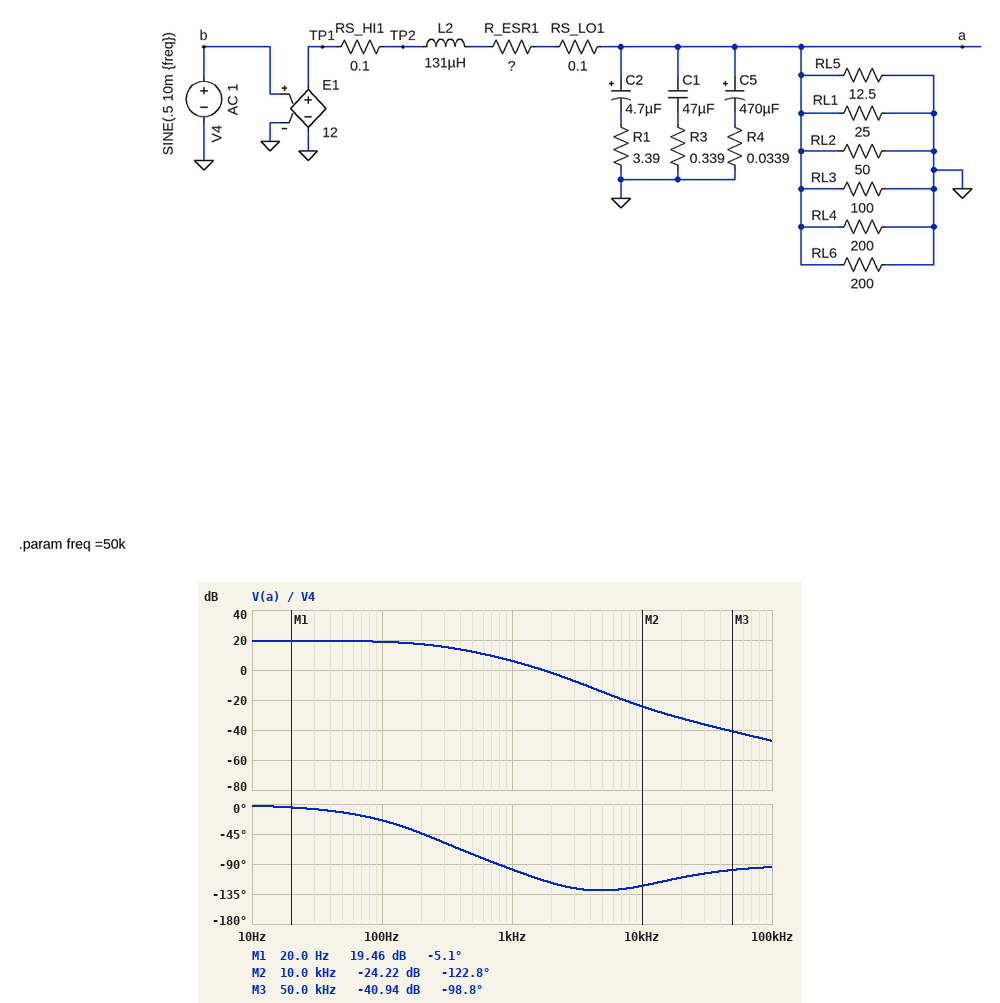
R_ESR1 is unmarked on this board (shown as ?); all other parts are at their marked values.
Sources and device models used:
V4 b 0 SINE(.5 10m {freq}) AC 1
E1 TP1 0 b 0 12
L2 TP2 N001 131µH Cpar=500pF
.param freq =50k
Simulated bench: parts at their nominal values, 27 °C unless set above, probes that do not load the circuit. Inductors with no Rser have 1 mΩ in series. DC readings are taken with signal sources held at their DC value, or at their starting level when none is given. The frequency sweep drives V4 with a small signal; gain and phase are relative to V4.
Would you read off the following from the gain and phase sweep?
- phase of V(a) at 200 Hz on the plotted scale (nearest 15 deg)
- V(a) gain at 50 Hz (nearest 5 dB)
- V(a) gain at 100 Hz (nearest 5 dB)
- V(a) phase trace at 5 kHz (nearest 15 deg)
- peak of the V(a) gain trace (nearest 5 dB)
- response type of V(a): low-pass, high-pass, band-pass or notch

-45 deg
20 dB
20 dB
-135 deg
20 dB
low-pass
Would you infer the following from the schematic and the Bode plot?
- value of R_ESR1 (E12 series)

1.5 Ω
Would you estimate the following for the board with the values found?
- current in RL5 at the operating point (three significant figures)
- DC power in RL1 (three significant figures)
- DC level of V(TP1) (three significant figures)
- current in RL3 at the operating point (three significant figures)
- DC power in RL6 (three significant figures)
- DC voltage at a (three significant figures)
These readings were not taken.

377 mA
890 mW
6.00 V
47.2 mA
111 mW
4.72 V
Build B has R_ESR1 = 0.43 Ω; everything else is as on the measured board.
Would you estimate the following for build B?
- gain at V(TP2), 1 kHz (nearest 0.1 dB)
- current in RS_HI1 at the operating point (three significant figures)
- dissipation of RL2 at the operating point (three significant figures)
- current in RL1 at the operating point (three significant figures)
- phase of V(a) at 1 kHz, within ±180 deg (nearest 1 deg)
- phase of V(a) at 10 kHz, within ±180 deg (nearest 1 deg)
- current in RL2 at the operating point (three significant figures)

20.8 dB
872 mA
594 mW
218 mA
-119 deg
-130 deg
109 mA
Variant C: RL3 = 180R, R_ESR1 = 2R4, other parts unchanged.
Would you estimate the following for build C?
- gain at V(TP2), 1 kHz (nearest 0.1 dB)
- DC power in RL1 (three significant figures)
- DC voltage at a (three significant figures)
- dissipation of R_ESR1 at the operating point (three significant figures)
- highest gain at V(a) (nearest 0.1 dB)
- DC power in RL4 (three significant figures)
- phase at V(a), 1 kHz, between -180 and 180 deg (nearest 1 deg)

21.3 dB
730 mW
4.27 V
1.06 W
18.6 dB
91.2 mW
-93 deg
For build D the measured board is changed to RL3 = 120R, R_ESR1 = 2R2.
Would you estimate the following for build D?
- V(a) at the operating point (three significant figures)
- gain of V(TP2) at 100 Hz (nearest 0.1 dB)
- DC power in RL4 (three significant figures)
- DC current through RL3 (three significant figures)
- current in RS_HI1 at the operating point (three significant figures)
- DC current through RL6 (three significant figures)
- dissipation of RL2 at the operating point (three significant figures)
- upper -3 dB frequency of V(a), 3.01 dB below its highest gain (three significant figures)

4.35 V
21.4 dB
94.5 mW
36.2 mA
688 mA
21.7 mA
378 mW
180 Hz
